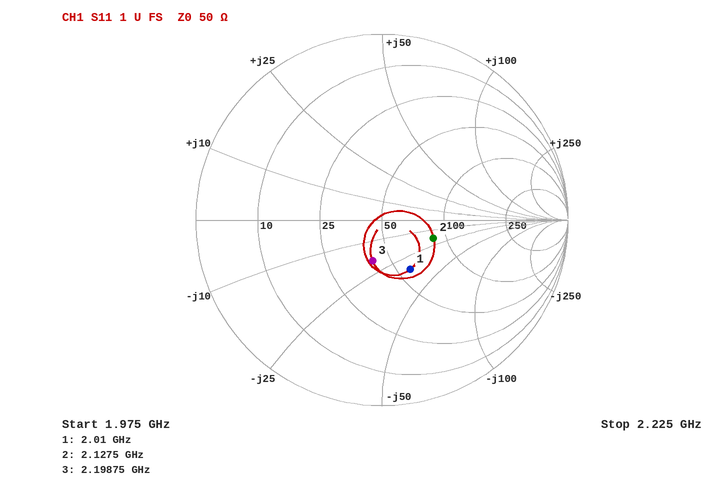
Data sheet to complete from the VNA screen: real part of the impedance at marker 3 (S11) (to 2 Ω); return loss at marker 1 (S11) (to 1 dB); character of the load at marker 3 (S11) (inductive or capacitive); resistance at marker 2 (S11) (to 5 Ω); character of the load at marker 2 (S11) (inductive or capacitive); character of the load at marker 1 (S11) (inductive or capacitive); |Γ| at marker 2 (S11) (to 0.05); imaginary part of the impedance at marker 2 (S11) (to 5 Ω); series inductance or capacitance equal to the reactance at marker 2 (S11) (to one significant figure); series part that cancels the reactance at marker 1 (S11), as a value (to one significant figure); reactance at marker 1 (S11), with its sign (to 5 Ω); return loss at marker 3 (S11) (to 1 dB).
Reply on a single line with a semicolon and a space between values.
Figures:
42 Ω; 10 dB; capacitive; 85 Ω; capacitive; capacitive; 0.30; -20 Ω; 4 pF; 3 nH; -35 Ω; 13 dB
